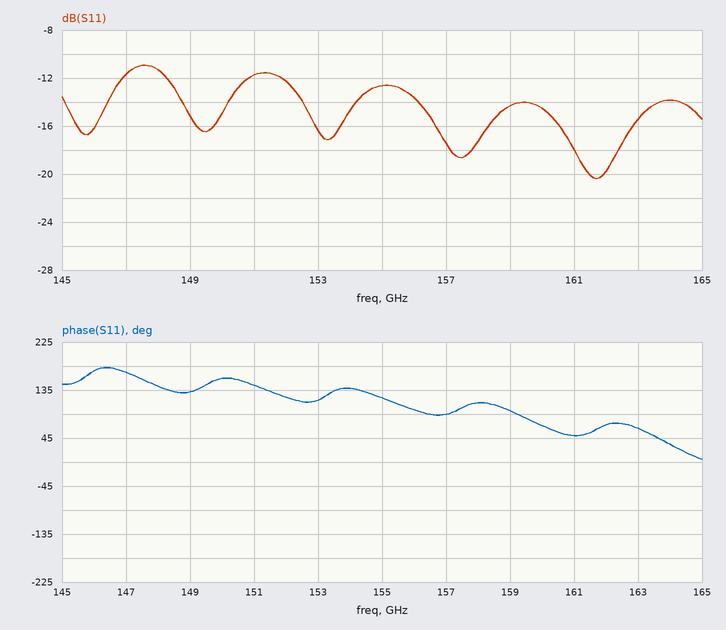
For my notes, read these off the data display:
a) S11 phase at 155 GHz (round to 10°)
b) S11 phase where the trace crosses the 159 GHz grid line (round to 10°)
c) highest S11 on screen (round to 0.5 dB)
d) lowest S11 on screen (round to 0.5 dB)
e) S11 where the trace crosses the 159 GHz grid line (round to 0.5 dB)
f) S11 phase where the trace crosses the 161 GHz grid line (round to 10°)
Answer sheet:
120°
100°
-11.0 dB
-20.5 dB
-14.5 dB
50°
